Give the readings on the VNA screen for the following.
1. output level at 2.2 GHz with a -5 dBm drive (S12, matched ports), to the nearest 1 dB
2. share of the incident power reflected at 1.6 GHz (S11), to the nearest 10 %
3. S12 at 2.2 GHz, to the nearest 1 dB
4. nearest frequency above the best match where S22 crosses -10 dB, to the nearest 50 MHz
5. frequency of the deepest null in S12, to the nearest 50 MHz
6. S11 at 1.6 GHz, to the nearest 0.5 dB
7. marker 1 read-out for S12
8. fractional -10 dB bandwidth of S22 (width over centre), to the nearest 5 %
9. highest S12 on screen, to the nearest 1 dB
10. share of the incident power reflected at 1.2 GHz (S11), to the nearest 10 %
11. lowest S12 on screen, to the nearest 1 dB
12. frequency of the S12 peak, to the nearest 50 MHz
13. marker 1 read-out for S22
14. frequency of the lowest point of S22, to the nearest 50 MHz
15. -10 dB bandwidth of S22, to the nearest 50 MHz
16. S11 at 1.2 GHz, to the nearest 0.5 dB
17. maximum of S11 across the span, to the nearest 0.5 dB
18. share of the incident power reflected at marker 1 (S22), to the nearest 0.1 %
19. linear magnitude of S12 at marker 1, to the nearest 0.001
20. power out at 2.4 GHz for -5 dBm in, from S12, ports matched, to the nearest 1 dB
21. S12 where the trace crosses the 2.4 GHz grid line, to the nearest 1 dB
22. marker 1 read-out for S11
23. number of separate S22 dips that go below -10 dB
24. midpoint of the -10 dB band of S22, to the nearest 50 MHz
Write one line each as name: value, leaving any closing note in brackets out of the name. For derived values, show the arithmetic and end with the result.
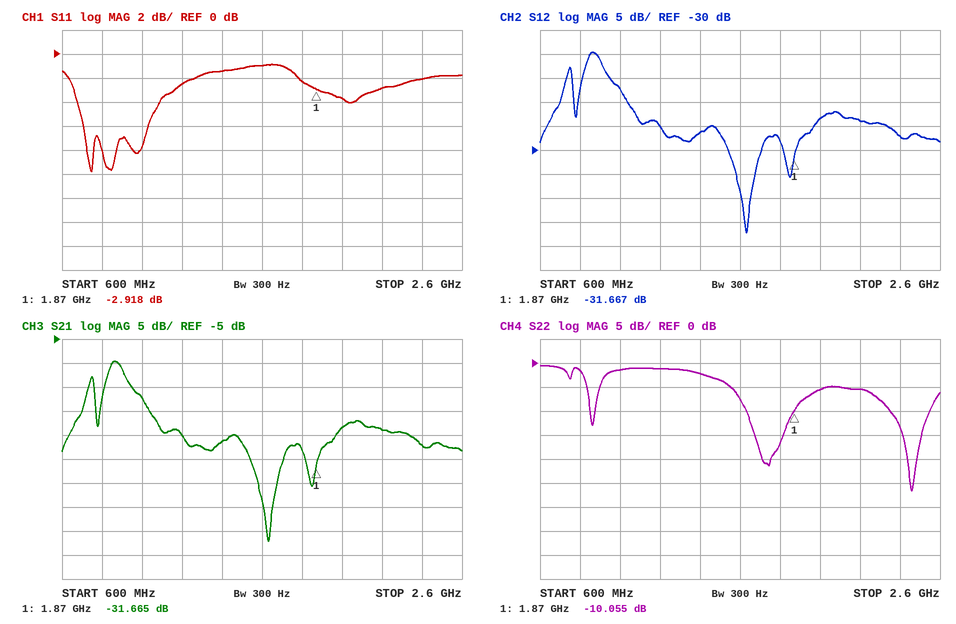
output level at 2.2 GHz with a -5 dBm drive (S12, matched ports), to the nearest 1 dB: -5 dBm + (-24 dB) = -29 dBm
share of the incident power reflected at 1.6 GHz (S11), to the nearest 10 %: 10^(-1/10) ≈ 79.4 %, so 80 % to the nearest 10 %
S12 at 2.2 GHz, to the nearest 1 dB: -24 dB
nearest frequency above the best match where S22 crosses -10 dB, to the nearest 50 MHz: 2.55 GHz
frequency of the deepest null in S12, to the nearest 50 MHz: 1.65 GHz
S11 at 1.6 GHz, to the nearest 0.5 dB: -1.0 dB
marker 1 read-out for S12: -31.667 dB
fractional -10 dB bandwidth of S22 (width over centre), to the nearest 5 %: 200 MHz / 2.45 GHz ≈ 8.16 %, so 10 % to the nearest 5 %
highest S12 on screen, to the nearest 1 dB: -10 dB
share of the incident power reflected at 1.2 GHz (S11), to the nearest 10 %: 10^(-2.5/10) ≈ 56.2 %, so 60 % to the nearest 10 %
lowest S12 on screen, to the nearest 1 dB: -47 dB
frequency of the S12 peak, to the nearest 50 MHz: 850 MHz
marker 1 read-out for S22: -10.055 dB
frequency of the lowest point of S22, to the nearest 50 MHz: 2.45 GHz
-10 dB bandwidth of S22, to the nearest 50 MHz: 2.55 GHz − 2.35 GHz = 200 MHz
S11 at 1.2 GHz, to the nearest 0.5 dB: -2.5 dB
maximum of S11 across the span, to the nearest 0.5 dB: -1.0 dB
share of the incident power reflected at marker 1 (S22), to the nearest 0.1 %: 10^(-10.055/10) ≈ 9.9 %
linear magnitude of S12 at marker 1, to the nearest 0.001: 10^(-31.667/20) ≈ 0.026
power out at 2.4 GHz for -5 dBm in, from S12, ports matched, to the nearest 1 dB: -5 dBm + (-27 dB) = -32 dBm
S12 where the trace crosses the 2.4 GHz grid line, to the nearest 1 dB: -27 dB
marker 1 read-out for S11: -2.918 dB
number of separate S22 dips that go below -10 dB: 3
midpoint of the -10 dB band of S22, to the nearest 50 MHz: 2.45 GHz
